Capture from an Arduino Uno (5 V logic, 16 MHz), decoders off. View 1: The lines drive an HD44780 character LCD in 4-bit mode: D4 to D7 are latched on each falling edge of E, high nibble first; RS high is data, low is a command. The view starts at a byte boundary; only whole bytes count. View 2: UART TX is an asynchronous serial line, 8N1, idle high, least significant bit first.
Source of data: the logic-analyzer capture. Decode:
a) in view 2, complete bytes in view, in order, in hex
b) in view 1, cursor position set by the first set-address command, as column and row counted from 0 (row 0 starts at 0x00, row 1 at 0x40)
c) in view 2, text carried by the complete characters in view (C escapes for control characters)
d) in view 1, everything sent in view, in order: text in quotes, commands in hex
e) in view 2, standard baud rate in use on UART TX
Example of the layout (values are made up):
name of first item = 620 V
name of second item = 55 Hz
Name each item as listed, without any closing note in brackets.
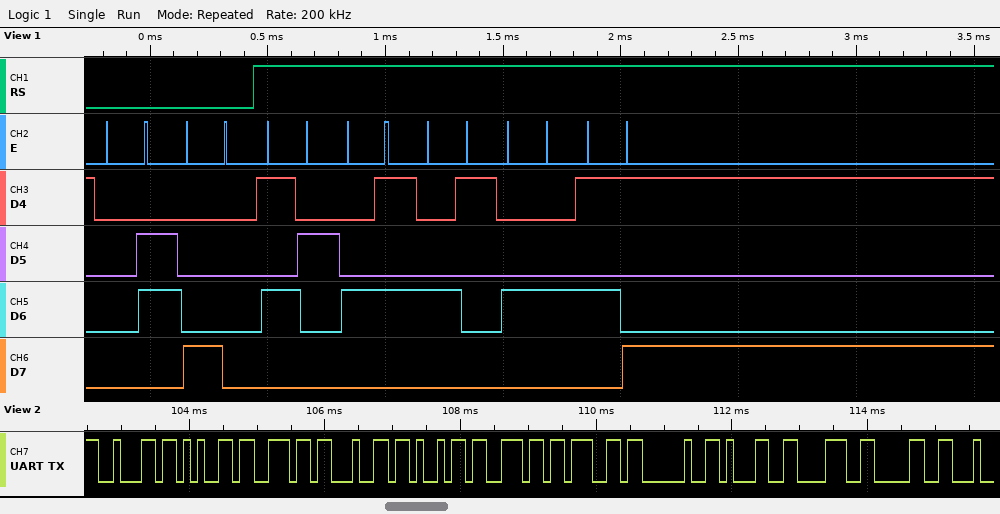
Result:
in view 2, complete bytes in view, in order, in hex = 62 65 6E 64 69 6E 67 20 31 38 30
in view 1, cursor position set by the first set-address command, as column and row counted from 0 = column 0, row 0
in view 2, text carried by the complete characters in view = "bending 180"
in view 1, everything sent in view, in order: text in quotes, commands in hex = 0x06 0x80 "READY"
in view 2, standard baud rate in use on UART TX = 9600 baud
